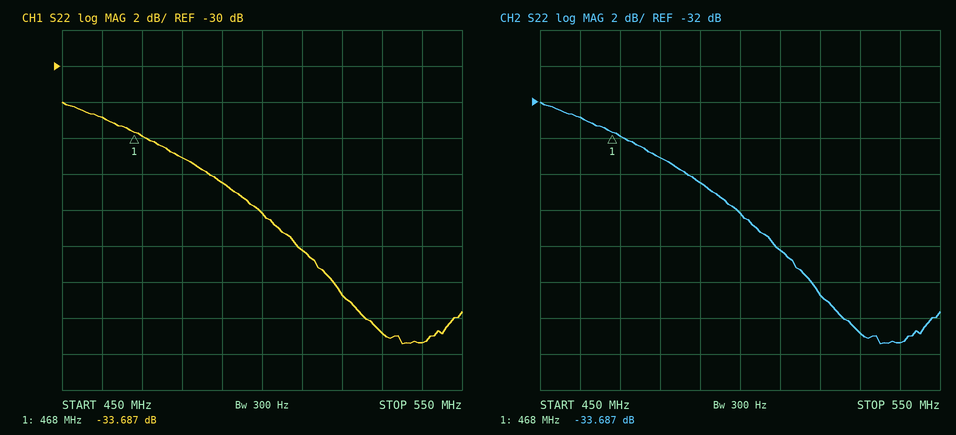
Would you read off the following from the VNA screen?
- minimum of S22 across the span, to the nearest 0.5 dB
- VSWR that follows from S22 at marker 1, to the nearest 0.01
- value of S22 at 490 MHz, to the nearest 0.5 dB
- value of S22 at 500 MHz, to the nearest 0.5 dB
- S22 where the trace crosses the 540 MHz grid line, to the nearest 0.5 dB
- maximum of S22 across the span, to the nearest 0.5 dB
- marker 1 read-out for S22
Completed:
-45.5 dB
1.04
-36.5 dB
-38.0 dB
-45.5 dB
-32.0 dB
-33.687 dB
